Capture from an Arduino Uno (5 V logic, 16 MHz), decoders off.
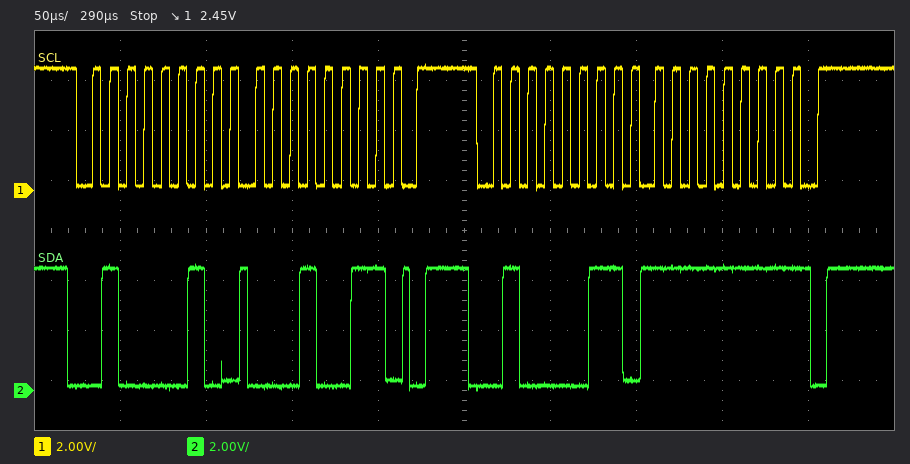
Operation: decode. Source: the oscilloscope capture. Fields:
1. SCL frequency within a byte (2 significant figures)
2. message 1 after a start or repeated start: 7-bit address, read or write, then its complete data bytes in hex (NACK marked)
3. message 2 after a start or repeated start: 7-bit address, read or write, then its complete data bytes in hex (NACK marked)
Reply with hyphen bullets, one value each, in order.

- 100 kHz
- 0x21 write: 13
- 0x21 read: FF NACK
